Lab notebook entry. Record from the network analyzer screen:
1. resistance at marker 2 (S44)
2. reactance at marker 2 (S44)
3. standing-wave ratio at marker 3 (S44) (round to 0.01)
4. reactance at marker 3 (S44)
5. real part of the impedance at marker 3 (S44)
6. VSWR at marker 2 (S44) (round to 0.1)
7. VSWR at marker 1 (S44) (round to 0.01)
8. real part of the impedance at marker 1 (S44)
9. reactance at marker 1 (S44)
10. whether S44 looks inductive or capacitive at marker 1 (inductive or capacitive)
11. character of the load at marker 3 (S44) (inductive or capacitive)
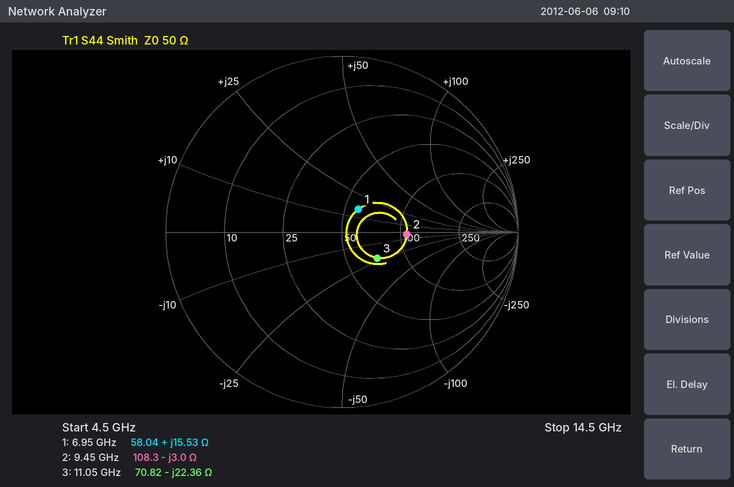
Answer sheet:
108.3 Ω
-3.0 Ω
1.66
-22.36 Ω
70.82 Ω
2.2
1.38
58.04 Ω
+15.53 Ω
inductive
capacitive
